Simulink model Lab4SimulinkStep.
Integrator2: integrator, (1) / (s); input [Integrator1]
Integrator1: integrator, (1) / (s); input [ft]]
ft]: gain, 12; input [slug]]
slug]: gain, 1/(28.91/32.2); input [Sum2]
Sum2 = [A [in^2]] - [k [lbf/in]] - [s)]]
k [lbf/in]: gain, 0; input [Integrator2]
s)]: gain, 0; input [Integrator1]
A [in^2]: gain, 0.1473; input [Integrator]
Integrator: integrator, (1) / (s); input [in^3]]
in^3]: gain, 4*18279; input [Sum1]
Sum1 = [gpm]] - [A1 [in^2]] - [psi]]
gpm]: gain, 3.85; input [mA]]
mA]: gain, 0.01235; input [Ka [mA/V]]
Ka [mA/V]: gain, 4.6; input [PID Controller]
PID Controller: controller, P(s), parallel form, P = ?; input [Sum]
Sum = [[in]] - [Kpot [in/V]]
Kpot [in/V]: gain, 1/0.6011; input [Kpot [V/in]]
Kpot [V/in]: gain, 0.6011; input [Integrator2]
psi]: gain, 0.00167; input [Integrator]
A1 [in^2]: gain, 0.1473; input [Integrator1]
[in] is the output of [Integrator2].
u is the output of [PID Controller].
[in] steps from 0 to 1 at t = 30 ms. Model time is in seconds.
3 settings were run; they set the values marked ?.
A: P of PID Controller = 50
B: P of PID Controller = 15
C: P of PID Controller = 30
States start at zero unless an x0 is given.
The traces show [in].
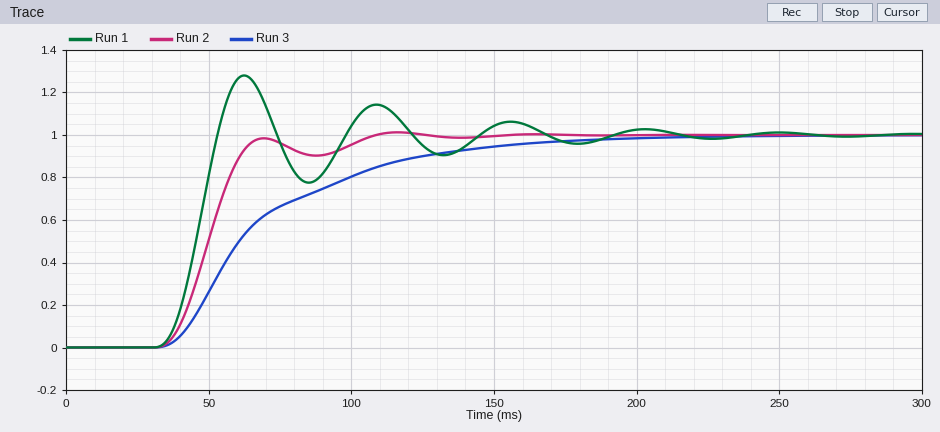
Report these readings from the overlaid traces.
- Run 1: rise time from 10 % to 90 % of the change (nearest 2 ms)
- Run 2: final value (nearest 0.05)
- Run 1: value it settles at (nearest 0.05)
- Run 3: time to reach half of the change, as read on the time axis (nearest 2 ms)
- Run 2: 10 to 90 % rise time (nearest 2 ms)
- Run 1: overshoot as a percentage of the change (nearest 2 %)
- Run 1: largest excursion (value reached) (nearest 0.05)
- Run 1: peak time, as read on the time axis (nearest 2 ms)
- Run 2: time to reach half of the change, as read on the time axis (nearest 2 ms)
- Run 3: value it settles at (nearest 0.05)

14 ms
1.00
1.00
60 ms
22 ms
28 %
1.30
62 ms
50 ms
1.00
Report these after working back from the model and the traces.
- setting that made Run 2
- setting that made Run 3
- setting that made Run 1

C
B
A
